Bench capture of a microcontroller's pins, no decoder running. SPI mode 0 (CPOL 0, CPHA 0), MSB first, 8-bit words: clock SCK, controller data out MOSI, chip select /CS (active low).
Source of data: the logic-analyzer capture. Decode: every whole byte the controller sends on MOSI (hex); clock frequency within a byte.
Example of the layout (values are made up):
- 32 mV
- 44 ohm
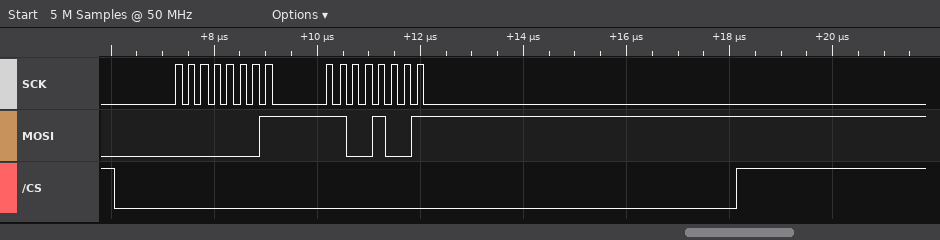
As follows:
- 01 C9
- 4 MHz
